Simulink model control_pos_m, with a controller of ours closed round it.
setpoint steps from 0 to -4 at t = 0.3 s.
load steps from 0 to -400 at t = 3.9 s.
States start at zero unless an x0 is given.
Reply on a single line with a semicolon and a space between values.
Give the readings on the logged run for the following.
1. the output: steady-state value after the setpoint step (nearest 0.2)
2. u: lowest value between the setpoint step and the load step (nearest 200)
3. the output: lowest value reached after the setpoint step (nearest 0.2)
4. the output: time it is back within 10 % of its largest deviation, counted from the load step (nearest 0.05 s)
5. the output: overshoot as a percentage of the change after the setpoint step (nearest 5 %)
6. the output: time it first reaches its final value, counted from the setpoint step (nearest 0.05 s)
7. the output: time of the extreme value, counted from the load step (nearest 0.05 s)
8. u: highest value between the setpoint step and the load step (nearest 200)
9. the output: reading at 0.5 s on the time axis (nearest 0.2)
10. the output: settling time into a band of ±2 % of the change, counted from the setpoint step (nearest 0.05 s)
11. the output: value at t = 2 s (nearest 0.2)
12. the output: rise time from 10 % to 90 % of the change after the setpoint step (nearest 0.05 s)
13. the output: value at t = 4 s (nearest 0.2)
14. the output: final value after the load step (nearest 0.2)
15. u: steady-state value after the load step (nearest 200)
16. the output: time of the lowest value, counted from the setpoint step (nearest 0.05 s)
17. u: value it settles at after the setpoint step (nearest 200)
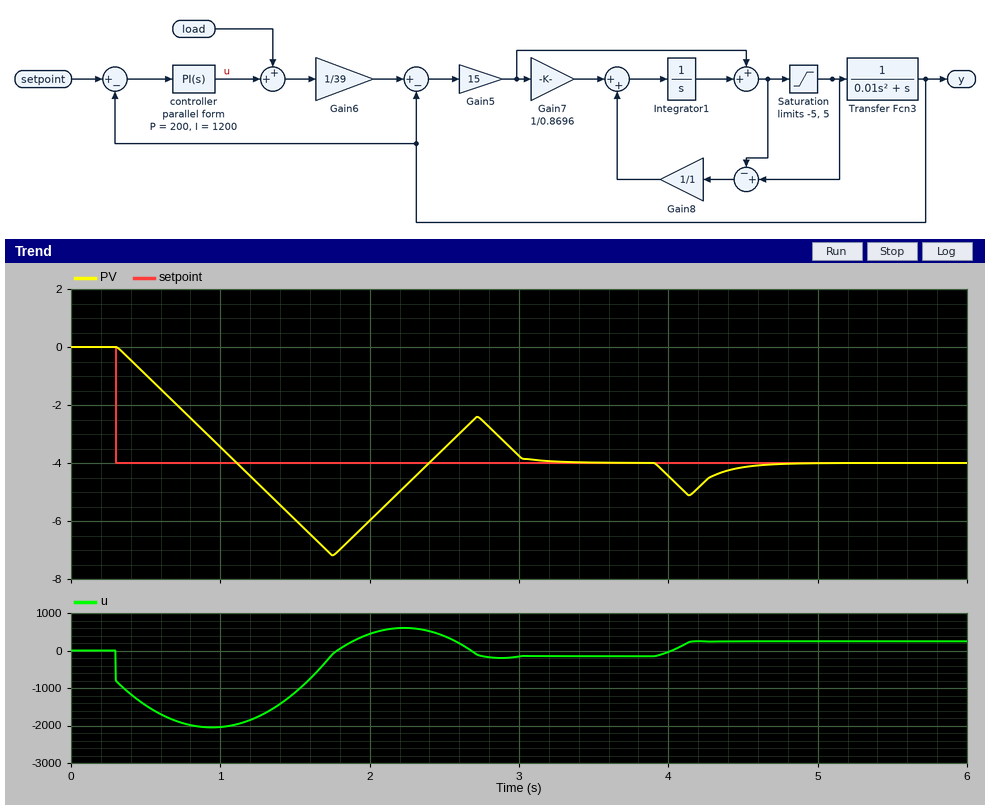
-4.0; -2000; -7.2; 0.65 s; 80 %; 0.80 s; 0.25 s; 600; -1.0; 2.85 s; -6.0; 0.65 s; -4.4; -4.0; 200; 1.45 s; -200
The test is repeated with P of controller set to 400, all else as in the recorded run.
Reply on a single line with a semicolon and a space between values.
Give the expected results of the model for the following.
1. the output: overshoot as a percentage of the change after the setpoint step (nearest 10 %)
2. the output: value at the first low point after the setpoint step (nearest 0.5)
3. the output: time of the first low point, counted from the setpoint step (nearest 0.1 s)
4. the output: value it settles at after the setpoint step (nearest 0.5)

70 %; -6.5; 1.3 s; -4.0
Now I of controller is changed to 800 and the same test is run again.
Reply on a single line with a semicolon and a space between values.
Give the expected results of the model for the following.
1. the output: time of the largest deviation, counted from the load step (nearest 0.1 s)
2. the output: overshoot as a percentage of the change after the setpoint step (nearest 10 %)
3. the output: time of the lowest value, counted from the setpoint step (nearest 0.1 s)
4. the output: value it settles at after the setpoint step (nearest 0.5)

0.3 s; 70 %; 1.4 s; -4.0
